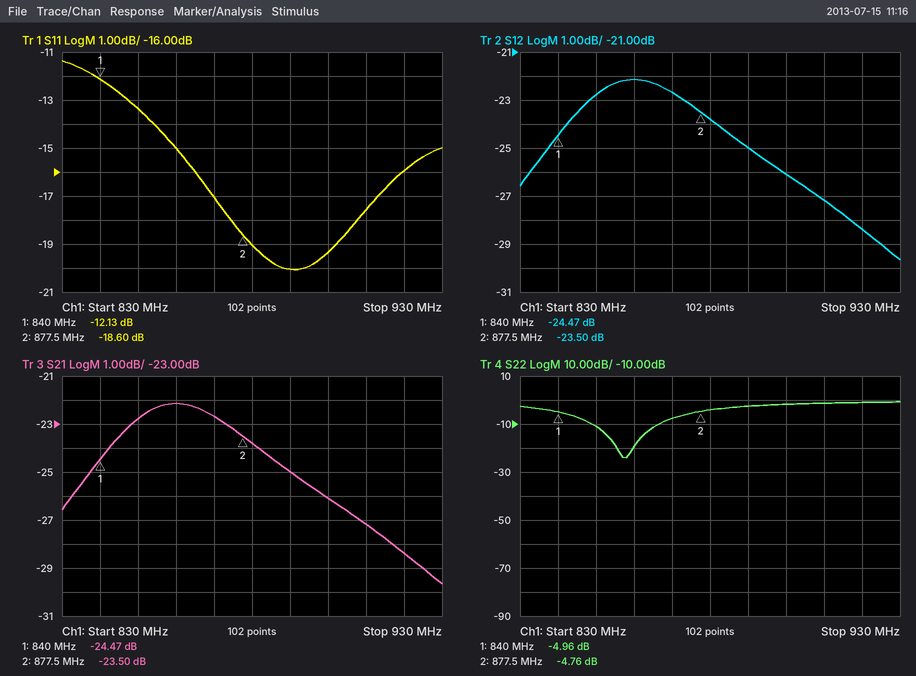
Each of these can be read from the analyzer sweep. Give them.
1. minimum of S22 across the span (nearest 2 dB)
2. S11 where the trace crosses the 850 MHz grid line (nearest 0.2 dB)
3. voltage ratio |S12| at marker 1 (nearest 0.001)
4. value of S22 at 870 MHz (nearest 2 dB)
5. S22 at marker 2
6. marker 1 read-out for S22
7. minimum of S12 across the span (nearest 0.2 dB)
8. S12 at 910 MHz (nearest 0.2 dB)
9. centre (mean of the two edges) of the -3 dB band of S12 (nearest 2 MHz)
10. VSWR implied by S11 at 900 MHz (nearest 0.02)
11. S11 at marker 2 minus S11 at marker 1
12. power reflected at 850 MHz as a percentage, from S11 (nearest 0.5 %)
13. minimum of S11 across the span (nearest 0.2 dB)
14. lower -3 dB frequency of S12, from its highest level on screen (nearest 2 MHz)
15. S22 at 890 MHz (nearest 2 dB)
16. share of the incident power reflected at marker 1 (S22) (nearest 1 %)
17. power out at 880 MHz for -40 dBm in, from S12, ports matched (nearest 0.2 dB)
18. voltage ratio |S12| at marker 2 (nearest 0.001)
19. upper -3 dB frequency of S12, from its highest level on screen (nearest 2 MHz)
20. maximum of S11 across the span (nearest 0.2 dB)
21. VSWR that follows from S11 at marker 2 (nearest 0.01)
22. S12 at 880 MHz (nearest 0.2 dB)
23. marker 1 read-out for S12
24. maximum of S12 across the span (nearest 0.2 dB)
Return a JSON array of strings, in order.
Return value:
["-24 dB", "-13.4 dB", "0.060", "-8 dB", "-4.76 dB", "-4.96 dB", "-29.6 dB", "-27.2 dB", "864 MHz", "1.24", "-6.47 dB", "4.5 %", "-20.0 dB", "836 MHz", "-2 dB", "32 %", "-63.8 dBm", "0.067", "892 MHz", "-11.4 dB", "1.27", "-23.8 dB", "-24.47 dB", "-22.2 dB"]
